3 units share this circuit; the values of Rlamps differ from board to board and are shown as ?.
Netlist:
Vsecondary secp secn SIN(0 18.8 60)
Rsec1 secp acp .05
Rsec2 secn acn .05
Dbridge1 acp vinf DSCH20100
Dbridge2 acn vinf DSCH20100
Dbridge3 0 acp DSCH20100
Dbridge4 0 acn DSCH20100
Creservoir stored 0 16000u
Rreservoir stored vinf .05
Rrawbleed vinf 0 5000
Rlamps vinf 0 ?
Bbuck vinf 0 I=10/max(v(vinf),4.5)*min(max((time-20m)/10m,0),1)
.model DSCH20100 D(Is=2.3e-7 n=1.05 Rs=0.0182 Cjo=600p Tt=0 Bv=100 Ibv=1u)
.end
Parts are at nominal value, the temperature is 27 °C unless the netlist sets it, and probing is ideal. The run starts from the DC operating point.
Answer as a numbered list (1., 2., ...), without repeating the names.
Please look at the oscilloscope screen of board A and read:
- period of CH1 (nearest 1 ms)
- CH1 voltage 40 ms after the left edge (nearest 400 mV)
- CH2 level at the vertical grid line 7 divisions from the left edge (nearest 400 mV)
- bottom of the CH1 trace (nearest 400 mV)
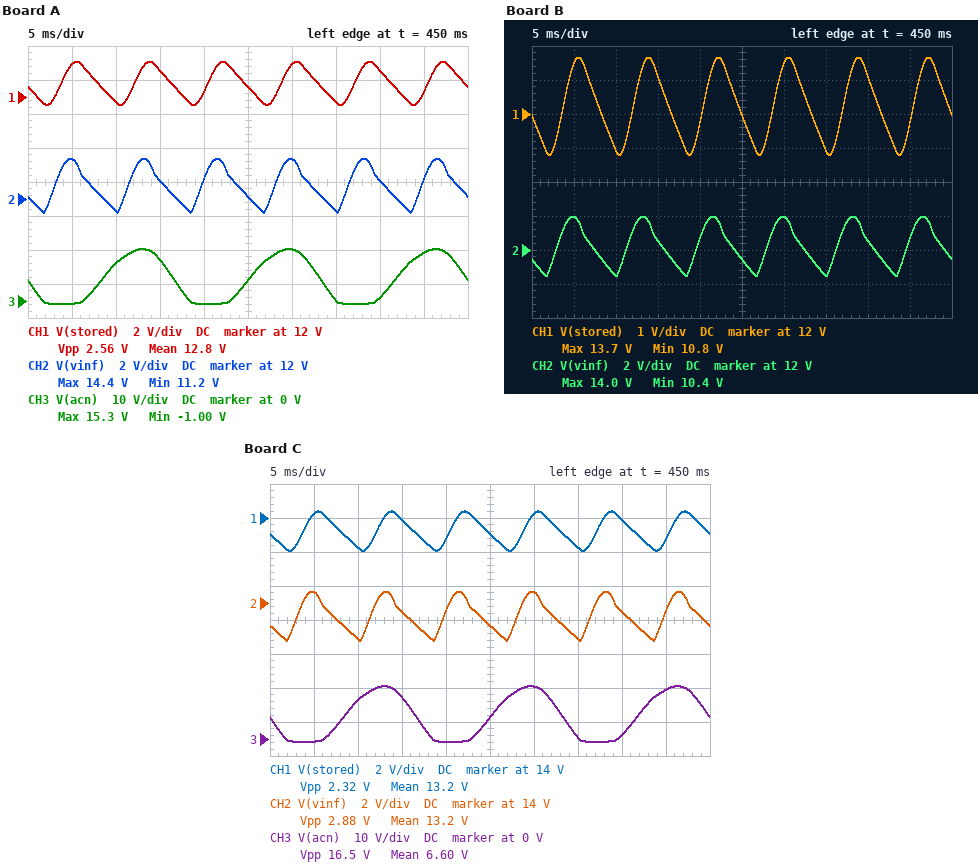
1. 8 ms
2. 13.6 V
3. 11.2 V
4. 11.6 V
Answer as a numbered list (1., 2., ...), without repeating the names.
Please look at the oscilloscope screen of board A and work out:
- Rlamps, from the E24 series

1. 1.5 Ω
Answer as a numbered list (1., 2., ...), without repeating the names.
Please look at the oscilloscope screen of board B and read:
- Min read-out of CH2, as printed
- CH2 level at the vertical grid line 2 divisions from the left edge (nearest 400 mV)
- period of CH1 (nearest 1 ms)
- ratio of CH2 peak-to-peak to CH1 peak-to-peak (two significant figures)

1. 10.4 V
2. 10.4 V
3. 8 ms
4. 1.2
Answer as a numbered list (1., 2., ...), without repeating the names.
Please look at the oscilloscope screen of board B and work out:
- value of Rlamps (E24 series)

1. 1.2 Ω
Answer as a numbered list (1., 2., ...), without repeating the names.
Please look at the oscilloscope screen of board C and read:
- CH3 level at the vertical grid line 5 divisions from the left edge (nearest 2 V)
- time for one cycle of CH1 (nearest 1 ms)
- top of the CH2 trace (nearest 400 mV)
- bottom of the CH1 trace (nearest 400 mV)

1. 6 V
2. 8 ms
3. 14.8 V
4. 12.0 V
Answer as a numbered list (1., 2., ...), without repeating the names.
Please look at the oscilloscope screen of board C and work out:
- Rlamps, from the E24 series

1. 1.8 Ω
